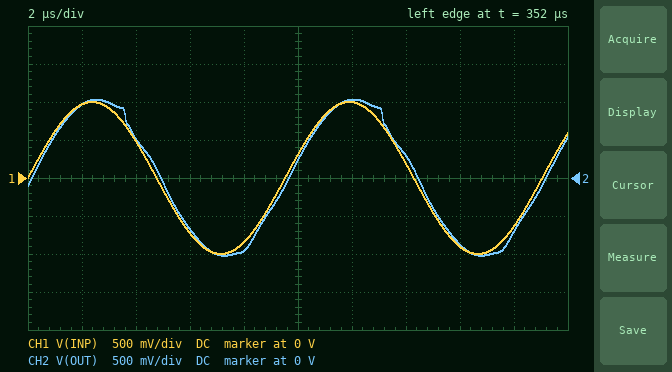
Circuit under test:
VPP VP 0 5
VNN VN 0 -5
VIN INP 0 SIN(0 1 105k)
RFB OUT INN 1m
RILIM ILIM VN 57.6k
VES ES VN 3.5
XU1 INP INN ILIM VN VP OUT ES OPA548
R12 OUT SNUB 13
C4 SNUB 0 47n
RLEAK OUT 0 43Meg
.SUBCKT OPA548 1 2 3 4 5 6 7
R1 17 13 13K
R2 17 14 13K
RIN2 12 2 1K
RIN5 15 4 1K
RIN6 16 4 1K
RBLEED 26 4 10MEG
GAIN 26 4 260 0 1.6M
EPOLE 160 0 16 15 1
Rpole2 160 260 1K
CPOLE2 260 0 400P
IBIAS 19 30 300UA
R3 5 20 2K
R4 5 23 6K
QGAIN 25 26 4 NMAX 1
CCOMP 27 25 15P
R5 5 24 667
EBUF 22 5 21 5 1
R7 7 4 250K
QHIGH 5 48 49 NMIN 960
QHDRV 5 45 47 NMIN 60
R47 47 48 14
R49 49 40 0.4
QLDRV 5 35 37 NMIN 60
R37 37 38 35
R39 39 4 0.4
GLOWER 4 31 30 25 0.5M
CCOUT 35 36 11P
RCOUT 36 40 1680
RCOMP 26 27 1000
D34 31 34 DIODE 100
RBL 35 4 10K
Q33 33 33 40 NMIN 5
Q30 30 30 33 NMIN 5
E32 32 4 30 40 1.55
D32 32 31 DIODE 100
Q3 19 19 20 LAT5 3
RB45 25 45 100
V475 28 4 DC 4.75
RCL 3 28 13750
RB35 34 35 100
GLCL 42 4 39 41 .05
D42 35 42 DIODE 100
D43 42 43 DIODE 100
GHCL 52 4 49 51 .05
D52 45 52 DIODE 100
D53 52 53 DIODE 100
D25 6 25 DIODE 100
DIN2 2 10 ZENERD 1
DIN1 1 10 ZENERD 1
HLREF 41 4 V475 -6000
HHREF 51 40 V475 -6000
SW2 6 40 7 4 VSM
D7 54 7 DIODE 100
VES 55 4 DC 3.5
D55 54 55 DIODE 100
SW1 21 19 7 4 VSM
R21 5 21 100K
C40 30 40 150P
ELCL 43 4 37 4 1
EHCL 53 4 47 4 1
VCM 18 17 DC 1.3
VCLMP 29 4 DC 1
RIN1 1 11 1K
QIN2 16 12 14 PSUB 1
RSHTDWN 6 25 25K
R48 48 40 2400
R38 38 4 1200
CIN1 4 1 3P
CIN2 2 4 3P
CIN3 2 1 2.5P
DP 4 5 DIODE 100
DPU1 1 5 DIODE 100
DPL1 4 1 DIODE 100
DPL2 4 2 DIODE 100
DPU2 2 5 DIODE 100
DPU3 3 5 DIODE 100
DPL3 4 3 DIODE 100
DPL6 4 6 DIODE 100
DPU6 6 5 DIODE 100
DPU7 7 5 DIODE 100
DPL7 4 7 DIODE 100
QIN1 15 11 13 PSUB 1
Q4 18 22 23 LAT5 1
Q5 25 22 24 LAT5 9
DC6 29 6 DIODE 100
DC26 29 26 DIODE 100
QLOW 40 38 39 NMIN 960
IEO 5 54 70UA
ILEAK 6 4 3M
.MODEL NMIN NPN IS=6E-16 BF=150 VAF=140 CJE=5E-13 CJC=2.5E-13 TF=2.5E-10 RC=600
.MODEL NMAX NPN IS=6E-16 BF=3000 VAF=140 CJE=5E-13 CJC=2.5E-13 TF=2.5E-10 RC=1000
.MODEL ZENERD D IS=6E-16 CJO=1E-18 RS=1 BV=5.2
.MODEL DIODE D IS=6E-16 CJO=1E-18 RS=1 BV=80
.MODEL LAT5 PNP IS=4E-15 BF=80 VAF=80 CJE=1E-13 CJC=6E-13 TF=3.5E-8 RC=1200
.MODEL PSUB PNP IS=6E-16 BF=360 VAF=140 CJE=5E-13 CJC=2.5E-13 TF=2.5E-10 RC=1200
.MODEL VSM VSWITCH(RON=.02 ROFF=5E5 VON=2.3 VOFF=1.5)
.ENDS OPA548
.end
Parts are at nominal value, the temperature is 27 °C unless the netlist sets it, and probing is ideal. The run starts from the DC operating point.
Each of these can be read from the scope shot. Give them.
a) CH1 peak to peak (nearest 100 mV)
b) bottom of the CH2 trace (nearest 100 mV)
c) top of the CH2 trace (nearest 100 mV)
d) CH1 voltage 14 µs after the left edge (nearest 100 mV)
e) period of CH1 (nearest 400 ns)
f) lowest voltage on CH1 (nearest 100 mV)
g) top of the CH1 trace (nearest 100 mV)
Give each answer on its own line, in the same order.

2.0 V
-1.0 V
1.0 V
200 mV
9.6 µs
-1.0 V
1.0 V
